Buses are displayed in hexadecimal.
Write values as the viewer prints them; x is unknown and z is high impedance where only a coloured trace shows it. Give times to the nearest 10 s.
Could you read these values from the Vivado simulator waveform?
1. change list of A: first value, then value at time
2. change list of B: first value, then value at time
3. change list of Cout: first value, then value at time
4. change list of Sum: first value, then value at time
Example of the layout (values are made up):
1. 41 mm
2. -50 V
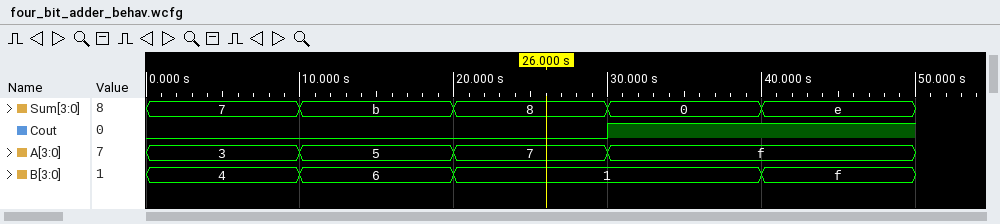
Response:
1. 3, 5 at 10 s, 7 at 20 s, f at 30 s
2. 4, 6 at 10 s, 1 at 20 s, f at 40 s
3. 0, 1 at 30 s
4. 7, b at 10 s, 8 at 20 s, 0 at 30 s, e at 40 s
